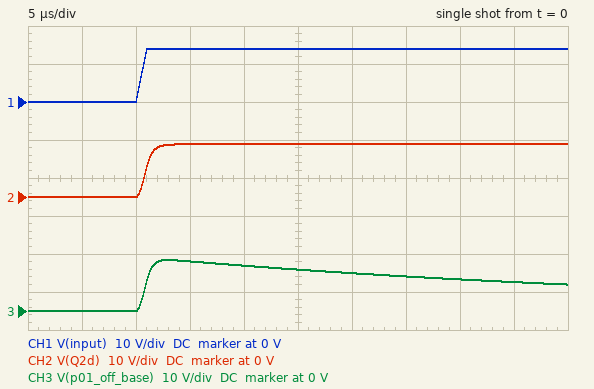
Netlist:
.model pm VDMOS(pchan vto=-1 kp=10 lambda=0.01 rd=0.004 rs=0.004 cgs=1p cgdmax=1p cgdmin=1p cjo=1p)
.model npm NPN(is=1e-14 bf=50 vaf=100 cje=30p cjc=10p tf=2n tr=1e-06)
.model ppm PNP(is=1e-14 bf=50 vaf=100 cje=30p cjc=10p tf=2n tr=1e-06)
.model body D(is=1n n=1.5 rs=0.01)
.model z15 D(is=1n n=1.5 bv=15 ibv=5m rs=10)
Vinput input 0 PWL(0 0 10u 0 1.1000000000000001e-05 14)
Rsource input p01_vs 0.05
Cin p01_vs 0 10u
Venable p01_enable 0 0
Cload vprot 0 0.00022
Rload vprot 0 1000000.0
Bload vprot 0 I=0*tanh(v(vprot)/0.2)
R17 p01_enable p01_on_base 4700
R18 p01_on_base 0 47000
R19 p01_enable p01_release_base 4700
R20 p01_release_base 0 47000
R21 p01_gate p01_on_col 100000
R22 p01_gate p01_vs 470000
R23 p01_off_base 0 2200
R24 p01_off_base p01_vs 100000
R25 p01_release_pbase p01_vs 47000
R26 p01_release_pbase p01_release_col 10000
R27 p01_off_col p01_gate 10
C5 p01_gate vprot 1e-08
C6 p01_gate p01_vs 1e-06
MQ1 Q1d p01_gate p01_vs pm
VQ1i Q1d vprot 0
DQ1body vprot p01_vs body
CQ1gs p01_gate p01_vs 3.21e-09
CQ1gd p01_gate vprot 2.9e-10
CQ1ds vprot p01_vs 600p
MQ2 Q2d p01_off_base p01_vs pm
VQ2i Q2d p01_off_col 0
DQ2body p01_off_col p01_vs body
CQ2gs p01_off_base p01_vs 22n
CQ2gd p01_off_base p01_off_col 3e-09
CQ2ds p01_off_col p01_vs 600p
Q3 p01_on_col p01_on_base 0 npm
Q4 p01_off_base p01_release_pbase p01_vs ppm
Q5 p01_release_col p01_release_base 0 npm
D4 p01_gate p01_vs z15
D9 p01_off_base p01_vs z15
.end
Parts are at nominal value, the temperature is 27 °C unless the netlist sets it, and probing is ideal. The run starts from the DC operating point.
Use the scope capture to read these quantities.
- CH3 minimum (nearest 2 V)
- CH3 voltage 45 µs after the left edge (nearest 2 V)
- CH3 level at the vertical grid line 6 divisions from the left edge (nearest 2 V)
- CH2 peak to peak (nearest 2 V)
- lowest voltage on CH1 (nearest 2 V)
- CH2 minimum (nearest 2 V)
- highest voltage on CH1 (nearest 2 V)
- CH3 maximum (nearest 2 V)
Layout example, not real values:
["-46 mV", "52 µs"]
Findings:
["0 V", "8 V", "10 V", "14 V", "0 V", "0 V", "14 V", "14 V"]
